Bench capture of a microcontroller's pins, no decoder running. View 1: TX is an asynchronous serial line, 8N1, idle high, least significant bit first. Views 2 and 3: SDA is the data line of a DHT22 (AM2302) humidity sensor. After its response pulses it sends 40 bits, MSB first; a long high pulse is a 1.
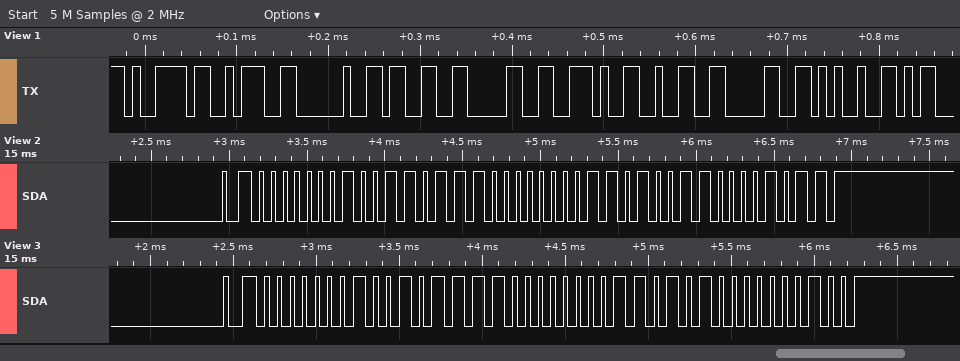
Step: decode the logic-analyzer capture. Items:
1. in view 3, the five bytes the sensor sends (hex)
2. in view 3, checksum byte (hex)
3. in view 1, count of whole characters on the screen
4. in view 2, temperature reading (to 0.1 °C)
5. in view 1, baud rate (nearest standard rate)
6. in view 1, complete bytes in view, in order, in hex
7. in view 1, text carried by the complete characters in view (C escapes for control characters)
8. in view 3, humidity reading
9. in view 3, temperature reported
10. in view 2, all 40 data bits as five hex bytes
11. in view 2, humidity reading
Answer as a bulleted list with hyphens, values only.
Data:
- 01 2F 00 D4 04
- 0x04
- 9
- 21.1 °C
- 115200 baud
- 0x79 0x3A 0x20 0x33 0x30 0x2E 0x32 0x30 0x25
- "y: 30.20%"
- 30.3 %
- 21.2 °C
- 01 37 00 D3 0B
- 31.1 %
